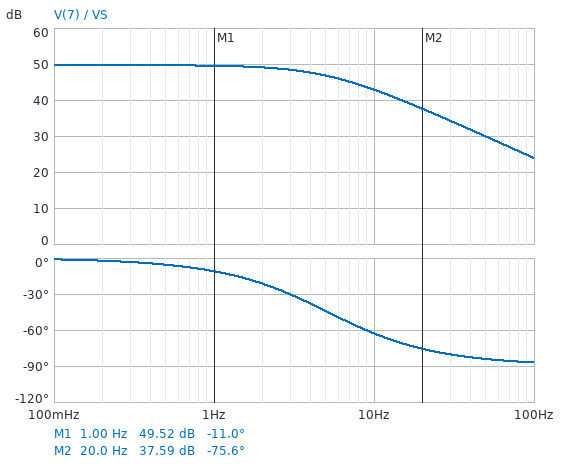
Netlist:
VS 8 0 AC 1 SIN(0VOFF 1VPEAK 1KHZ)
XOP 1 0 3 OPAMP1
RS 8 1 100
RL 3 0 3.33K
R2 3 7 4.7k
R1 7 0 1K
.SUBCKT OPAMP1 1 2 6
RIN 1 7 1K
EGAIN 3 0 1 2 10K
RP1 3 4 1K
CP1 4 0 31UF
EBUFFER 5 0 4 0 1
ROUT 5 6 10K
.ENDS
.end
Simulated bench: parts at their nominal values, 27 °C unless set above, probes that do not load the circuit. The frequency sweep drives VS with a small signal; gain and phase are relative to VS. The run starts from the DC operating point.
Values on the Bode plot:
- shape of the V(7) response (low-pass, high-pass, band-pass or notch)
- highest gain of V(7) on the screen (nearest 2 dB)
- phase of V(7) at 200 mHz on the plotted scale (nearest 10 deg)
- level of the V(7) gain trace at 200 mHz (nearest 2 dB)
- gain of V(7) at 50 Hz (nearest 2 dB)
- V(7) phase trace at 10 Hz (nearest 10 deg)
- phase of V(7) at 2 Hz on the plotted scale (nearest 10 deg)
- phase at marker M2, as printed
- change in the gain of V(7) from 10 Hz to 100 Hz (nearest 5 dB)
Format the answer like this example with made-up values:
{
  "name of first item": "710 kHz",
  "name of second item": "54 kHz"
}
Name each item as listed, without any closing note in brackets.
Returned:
{
  "shape of the V(7) response": "low-pass",
  "highest gain of V(7) on the screen": "50 dB",
  "phase of V(7) at 200 mHz on the plotted scale": "0 deg",
  "level of the V(7) gain trace at 200 mHz": "50 dB",
  "gain of V(7) at 50 Hz": "30 dB",
  "V(7) phase trace at 10 Hz": "-60 deg",
  "phase of V(7) at 2 Hz on the plotted scale": "-20 deg",
  "phase at marker M2, as printed": "-75.6 deg",
  "change in the gain of V(7) from 10 Hz to 100 Hz": "-20 dB"
}
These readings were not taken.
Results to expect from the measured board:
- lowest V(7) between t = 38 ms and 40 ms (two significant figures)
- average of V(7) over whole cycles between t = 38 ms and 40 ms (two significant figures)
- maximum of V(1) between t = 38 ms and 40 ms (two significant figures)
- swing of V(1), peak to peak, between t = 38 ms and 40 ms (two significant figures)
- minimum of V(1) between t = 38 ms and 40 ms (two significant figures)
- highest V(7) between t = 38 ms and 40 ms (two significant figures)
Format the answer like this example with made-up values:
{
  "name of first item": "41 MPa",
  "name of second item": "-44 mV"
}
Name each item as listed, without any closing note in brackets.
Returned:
{
  "lowest V(7) between t = 38 ms and 40 ms": "-1.1 V",
  "average of V(7) over whole cycles between t = 38 ms and 40 ms": "450 mV",
  "maximum of V(1) between t = 38 ms and 40 ms": "1.0 V",
  "swing of V(1), peak to peak, between t = 38 ms and 40 ms": "2.0 V",
  "minimum of V(1) between t = 38 ms and 40 ms": "-1.0 V",
  "highest V(7) between t = 38 ms and 40 ms": "2.0 V"
}
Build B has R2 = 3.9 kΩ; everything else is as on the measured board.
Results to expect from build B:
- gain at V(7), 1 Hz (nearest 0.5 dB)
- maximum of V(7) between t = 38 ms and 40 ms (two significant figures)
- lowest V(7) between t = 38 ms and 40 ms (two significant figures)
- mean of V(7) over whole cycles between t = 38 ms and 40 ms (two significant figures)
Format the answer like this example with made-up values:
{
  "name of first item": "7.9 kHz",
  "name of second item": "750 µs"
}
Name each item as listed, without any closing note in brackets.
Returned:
{
  "gain at V(7), 1 Hz": "50.5 dB",
  "maximum of V(7) between t = 38 ms and 40 ms": "2.2 V",
  "lowest V(7) between t = 38 ms and 40 ms": "-1.3 V",
  "mean of V(7) over whole cycles between t = 38 ms and 40 ms": "500 mV"
}
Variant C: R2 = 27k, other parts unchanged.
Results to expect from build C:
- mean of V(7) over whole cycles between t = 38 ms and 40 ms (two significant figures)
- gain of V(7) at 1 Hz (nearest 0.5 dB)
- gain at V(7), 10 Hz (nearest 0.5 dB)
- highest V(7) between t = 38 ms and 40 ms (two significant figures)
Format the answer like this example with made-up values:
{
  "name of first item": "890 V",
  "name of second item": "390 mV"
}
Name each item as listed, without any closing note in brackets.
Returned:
{
  "mean of V(7) over whole cycles between t = 38 ms and 40 ms": "120 mV",
  "gain of V(7) at 1 Hz": "38.0 dB",
  "gain at V(7), 10 Hz": "31.5 dB",
  "highest V(7) between t = 38 ms and 40 ms": "540 mV"
}
